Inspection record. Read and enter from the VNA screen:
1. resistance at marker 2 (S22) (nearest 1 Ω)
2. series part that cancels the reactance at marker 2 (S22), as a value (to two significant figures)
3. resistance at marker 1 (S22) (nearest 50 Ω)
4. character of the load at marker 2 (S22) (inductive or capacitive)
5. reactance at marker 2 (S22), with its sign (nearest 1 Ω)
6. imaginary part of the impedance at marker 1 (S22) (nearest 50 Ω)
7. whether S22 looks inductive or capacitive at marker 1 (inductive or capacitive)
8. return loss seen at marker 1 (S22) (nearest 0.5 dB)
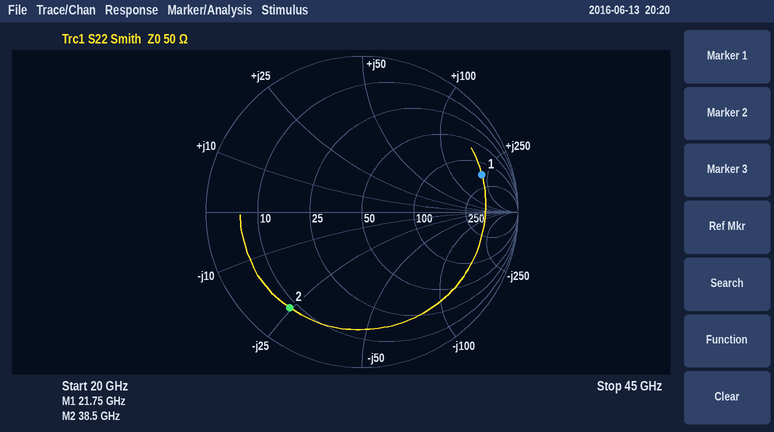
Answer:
8 Ω
100 pH
150 Ω
capacitive
-24 Ω
+200 Ω
inductive
2.0 dB
